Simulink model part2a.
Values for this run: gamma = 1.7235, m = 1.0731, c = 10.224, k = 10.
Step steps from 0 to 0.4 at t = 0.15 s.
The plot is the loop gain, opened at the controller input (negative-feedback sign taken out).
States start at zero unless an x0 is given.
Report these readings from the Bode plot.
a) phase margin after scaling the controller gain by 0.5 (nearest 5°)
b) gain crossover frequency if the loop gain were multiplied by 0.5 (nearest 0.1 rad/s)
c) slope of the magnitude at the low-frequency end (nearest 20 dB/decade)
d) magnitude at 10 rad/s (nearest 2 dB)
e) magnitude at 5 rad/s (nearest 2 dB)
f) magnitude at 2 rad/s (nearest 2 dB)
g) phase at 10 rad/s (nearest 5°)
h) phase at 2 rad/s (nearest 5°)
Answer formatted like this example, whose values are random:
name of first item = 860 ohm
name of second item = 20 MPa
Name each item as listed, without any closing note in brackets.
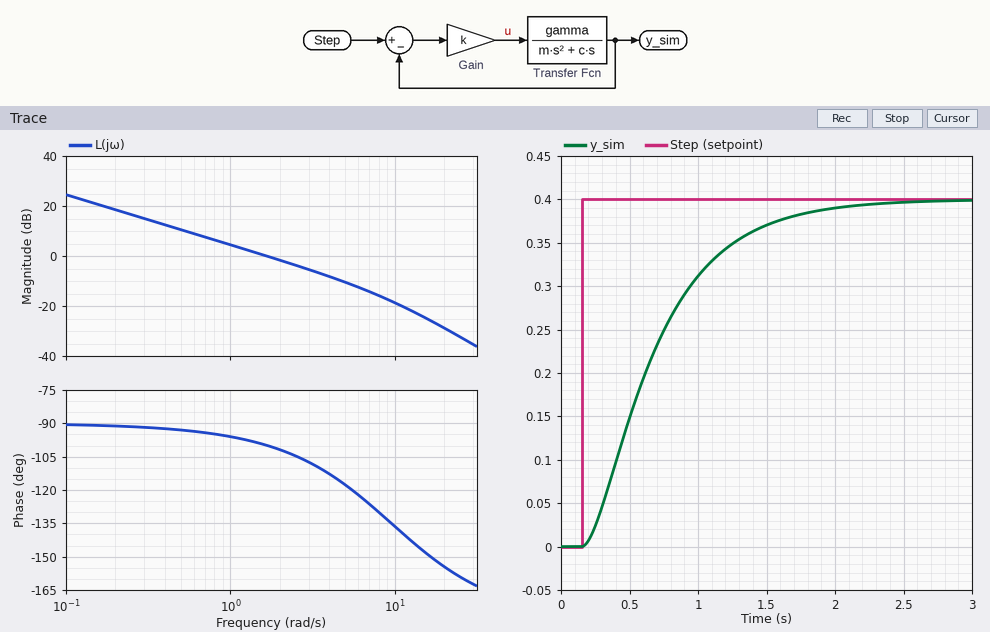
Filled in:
phase margin after scaling the controller gain by 0.5 = 85°
gain crossover frequency if the loop gain were multiplied by 0.5 = 0.8 rad/s
slope of the magnitude at the low-frequency end = -20 dB/decade
magnitude at 10 rad/s = -18 dB
magnitude at 5 rad/s = -10 dB
magnitude at 2 rad/s = -2 dB
phase at 10 rad/s = -135°
phase at 2 rad/s = -100°
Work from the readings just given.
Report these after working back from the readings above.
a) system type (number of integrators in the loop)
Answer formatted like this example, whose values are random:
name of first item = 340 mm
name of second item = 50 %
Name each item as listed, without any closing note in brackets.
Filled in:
system type = 1
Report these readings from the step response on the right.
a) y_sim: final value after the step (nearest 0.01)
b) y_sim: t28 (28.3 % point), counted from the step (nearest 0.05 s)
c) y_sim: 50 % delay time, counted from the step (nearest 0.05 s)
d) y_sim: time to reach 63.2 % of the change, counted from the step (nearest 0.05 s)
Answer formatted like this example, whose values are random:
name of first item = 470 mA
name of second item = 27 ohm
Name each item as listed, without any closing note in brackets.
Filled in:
y_sim: final value after the step = 0.40
y_sim: t28 (28.3 % point), counted from the step = 0.30 s
y_sim: 50 % delay time, counted from the step = 0.45 s
y_sim: time to reach 63.2 % of the change, counted from the step = 0.60 s
